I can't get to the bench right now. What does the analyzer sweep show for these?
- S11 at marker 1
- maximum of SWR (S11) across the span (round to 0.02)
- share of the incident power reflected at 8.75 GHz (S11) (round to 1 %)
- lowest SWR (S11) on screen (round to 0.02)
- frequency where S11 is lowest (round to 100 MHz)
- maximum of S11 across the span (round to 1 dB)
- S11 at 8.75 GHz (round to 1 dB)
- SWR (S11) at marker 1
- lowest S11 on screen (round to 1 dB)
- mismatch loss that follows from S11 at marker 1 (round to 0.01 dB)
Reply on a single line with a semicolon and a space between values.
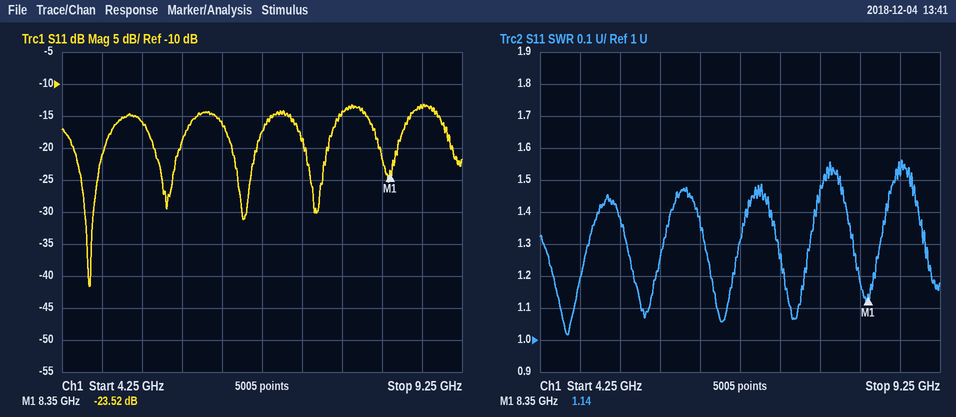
-23.52 dB; 1.56; 4 %; 1.02; 4.6 GHz; -13 dB; -14 dB; 1.14; -42 dB; 0.02 dB
